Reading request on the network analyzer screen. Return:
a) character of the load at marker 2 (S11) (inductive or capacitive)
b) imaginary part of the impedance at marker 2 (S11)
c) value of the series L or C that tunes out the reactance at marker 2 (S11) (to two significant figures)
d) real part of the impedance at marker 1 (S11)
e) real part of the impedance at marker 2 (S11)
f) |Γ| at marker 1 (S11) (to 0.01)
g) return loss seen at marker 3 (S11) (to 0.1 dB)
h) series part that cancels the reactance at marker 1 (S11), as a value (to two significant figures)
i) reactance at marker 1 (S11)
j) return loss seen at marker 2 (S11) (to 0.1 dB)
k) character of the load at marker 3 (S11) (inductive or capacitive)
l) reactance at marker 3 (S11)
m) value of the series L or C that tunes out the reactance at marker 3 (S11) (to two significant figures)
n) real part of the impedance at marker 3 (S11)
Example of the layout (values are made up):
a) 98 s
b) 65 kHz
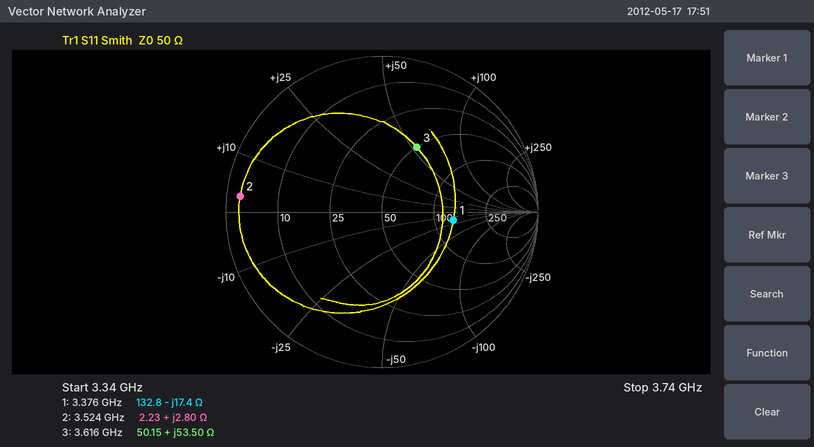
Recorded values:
a) inductive
b) +2.80 Ω
c) 16 pF
d) 132.8 Ω
e) 2.23 Ω
f) 0.46
g) 6.5 dB
h) 820 pH
i) -17.4 Ω
j) 0.8 dB
k) inductive
l) +53.50 Ω
m) 820 fF
n) 50.15 Ω
